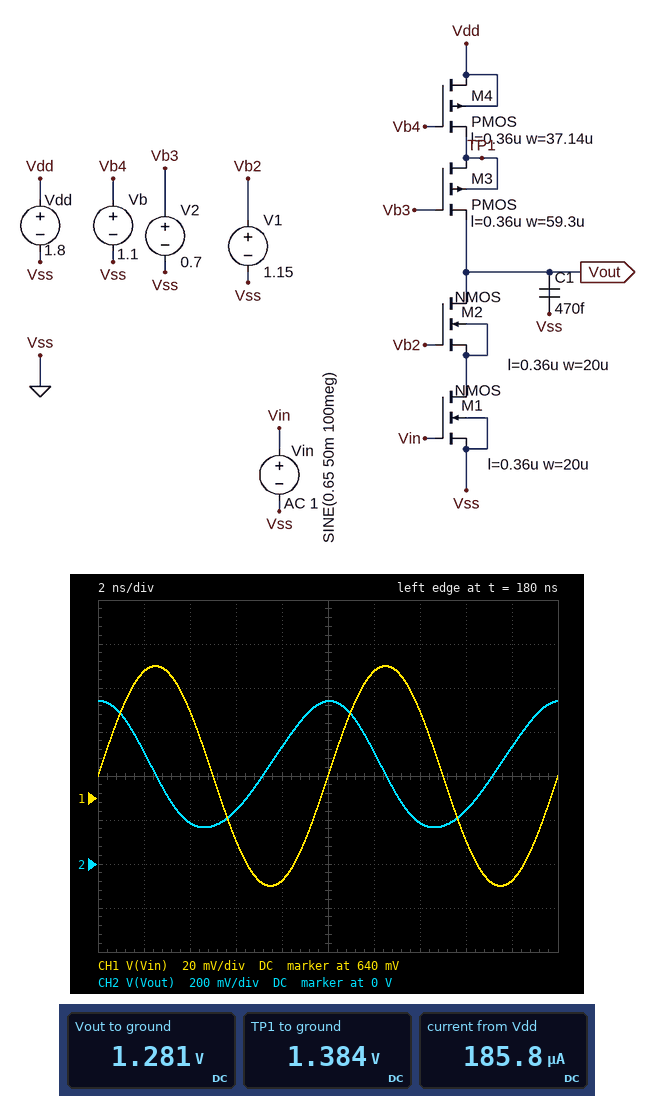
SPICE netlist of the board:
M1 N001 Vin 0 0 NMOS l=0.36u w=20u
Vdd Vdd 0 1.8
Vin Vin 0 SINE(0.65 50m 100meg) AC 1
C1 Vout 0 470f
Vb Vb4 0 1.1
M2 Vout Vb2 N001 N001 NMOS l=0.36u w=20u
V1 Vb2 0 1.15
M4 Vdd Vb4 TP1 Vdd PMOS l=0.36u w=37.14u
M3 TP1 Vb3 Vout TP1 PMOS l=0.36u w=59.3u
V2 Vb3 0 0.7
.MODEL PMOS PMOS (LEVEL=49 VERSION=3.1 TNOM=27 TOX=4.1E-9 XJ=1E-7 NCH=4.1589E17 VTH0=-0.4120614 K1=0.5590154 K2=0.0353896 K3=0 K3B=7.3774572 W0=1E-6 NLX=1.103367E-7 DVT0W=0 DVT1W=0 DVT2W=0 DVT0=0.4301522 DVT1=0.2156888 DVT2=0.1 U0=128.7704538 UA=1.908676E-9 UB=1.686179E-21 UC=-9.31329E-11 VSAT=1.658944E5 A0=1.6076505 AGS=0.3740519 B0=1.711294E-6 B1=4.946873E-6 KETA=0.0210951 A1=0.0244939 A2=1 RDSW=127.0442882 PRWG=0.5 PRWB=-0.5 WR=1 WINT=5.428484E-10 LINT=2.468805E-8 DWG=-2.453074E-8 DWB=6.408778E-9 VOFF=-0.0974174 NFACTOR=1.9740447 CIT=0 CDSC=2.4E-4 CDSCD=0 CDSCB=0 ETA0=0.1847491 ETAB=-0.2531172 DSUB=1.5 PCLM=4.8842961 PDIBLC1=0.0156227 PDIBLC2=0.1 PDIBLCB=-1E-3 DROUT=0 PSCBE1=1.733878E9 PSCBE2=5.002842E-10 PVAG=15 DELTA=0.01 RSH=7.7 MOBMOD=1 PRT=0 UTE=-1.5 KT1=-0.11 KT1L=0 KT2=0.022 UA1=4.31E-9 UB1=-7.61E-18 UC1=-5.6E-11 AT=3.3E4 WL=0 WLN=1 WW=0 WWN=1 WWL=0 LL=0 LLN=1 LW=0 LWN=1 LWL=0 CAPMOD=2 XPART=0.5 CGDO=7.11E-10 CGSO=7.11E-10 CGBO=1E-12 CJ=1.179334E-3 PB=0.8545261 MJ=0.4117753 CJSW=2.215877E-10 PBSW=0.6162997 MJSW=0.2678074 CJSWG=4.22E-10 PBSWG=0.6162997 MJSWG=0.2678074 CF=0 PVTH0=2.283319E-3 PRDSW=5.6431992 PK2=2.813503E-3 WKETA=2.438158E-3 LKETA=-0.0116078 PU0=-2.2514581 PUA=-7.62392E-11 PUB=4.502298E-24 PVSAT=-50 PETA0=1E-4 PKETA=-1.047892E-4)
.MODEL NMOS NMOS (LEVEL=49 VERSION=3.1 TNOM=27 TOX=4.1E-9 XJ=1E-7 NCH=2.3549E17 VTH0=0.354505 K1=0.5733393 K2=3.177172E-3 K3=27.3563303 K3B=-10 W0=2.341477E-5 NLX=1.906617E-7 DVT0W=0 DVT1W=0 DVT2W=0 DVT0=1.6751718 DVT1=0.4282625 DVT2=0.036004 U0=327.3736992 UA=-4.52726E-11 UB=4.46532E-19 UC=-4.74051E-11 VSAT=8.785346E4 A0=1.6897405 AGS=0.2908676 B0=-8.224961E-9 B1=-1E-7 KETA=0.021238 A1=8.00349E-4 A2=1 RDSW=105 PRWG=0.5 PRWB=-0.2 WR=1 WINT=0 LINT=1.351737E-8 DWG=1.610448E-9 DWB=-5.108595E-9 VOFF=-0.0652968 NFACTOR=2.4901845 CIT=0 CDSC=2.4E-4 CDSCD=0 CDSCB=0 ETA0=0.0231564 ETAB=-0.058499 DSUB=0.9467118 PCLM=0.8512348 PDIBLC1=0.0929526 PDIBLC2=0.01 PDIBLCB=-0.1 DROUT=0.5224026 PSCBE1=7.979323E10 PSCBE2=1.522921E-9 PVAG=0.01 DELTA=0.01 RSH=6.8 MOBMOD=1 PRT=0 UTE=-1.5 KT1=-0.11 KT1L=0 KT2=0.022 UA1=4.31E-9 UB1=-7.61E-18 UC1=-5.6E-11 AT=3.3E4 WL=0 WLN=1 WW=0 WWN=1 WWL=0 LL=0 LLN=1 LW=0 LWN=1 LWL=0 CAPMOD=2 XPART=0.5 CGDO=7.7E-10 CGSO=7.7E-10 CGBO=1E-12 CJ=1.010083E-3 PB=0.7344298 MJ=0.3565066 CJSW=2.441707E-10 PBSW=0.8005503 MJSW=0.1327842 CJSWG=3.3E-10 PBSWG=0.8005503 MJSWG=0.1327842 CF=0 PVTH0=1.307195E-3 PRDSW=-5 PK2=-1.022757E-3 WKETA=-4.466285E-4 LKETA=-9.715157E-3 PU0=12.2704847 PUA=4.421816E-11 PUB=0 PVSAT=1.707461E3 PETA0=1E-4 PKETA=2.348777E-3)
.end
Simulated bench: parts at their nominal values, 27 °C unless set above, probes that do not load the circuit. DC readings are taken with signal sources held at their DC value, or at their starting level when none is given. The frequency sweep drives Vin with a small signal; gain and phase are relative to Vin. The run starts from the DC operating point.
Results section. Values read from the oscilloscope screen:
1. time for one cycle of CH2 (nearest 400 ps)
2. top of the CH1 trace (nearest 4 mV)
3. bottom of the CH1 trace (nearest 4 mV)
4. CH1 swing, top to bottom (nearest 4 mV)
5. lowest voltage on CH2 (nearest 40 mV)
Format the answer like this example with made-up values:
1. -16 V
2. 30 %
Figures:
1. 10.0 ns
2. 700 mV
3. 600 mV
4. 100 mV
5. 160 mV
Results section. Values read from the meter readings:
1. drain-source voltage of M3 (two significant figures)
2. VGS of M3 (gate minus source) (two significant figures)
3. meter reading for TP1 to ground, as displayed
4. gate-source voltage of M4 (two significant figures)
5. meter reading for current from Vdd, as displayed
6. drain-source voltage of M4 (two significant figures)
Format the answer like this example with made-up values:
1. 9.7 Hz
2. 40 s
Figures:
1. 100 mV
2. -580 mV
3. 1.384 V
4. -280 mV
5. 185.8 µA
6. 420 mV
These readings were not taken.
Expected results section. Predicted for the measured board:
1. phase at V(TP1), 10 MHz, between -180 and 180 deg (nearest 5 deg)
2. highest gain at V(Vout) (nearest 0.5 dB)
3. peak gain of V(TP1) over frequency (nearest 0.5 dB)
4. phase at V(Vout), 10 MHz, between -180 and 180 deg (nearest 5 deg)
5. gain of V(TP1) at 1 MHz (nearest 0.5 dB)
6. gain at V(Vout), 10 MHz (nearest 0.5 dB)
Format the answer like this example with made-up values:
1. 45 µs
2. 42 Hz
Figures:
1. 105 deg
2. 47.0 dB
3. 41.0 dB
4. 105 deg
5. 40.0 dB
6. 34.5 dB
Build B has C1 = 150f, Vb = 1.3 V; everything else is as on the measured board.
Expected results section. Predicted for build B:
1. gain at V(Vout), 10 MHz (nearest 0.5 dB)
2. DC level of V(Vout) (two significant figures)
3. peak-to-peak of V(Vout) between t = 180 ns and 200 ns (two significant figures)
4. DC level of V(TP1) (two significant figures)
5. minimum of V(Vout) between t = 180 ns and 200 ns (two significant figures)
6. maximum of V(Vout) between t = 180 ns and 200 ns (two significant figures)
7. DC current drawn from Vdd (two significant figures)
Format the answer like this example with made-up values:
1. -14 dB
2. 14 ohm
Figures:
1. -27.0 dB
2. 7.3 mV
3. 5.2 mV
4. 1.2 V
5. 5.6 mV
6. 11 mV
7. 13 µA
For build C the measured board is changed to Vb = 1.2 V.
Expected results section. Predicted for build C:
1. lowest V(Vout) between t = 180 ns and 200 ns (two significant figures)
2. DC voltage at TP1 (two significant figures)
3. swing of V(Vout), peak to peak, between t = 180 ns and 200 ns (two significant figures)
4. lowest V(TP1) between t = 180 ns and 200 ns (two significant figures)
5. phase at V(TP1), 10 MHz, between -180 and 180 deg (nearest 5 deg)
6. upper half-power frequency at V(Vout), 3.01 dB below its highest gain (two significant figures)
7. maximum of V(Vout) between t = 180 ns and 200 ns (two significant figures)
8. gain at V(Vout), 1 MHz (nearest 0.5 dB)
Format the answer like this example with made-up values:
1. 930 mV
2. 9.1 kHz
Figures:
1. 31 mV
2. 1.3 V
3. 39 mV
4. 1.3 V
5. -170 deg
6. 370 MHz
7. 71 mV
8. -9.5 dB
